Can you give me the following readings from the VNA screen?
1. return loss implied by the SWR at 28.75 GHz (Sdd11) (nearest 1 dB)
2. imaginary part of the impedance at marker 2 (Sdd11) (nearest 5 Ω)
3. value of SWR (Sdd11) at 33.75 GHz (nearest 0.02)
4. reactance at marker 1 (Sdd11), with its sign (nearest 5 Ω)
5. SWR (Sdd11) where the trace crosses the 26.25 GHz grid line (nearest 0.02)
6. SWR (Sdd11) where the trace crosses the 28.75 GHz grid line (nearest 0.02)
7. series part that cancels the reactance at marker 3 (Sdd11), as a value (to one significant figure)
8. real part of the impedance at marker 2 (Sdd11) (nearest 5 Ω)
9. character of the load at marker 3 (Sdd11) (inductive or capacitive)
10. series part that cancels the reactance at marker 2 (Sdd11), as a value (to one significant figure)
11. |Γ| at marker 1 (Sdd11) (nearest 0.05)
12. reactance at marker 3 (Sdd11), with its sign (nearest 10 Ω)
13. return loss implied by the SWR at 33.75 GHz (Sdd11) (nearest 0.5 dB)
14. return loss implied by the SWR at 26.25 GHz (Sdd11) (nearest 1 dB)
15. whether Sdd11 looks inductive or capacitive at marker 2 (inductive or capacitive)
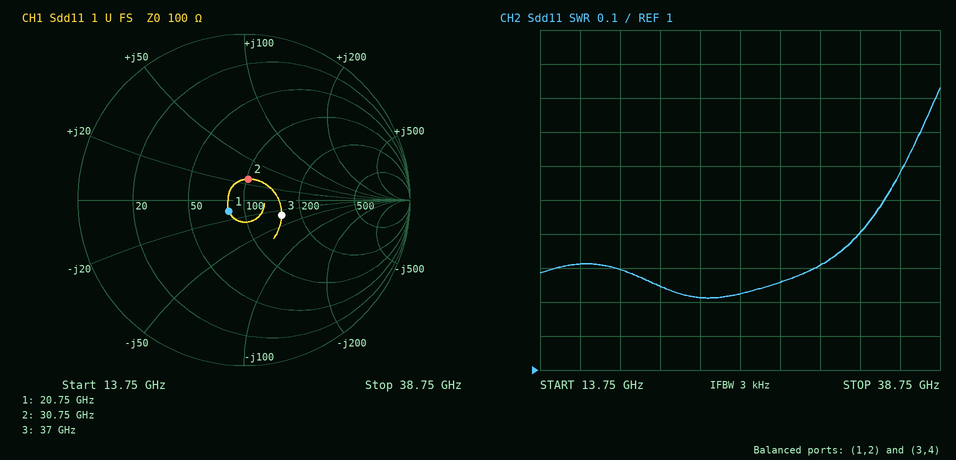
19 dB
+25 Ω
1.40
-10 Ω
1.22
1.26
100 pH
100 Ω
capacitive
200 fF
0.10
-30 Ω
15.5 dB
20 dB
inductive
